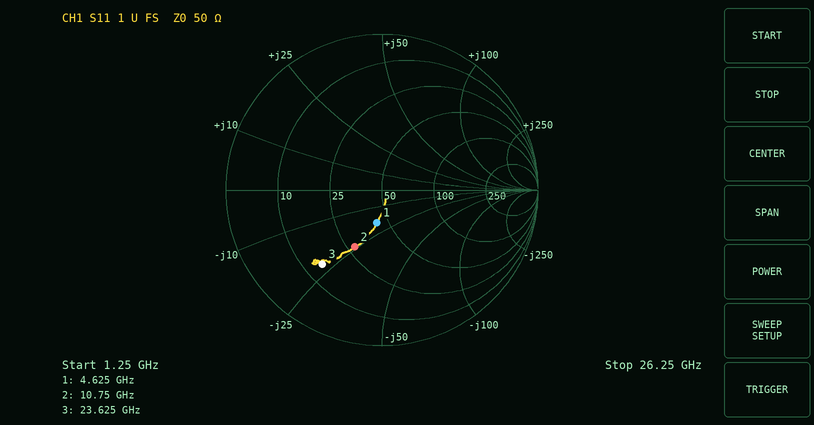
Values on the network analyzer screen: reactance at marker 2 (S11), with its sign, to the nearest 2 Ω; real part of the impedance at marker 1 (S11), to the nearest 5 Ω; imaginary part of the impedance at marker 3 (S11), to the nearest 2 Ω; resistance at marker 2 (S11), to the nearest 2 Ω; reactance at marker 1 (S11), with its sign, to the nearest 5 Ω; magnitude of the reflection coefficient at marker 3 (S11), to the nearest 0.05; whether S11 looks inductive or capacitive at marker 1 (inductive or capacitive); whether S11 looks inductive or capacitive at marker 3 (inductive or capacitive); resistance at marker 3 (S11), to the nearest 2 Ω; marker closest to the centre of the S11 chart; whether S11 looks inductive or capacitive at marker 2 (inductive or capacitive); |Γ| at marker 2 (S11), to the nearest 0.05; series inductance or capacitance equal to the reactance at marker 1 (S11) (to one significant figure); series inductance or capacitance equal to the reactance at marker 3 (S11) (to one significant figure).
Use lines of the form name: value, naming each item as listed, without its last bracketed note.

reactance at marker 2 (S11), with its sign, to the nearest 2 Ω: -24 Ω
real part of the impedance at marker 1 (S11), to the nearest 5 Ω: 45 Ω
imaginary part of the impedance at marker 3 (S11), to the nearest 2 Ω: -22 Ω
resistance at marker 2 (S11), to the nearest 2 Ω: 28 Ω
reactance at marker 1 (S11), with its sign, to the nearest 5 Ω: -20 Ω
magnitude of the reflection coefficient at marker 3 (S11), to the nearest 0.05: 0.60
whether S11 looks inductive or capacitive at marker 1: capacitive
whether S11 looks inductive or capacitive at marker 3: capacitive
resistance at marker 3 (S11), to the nearest 2 Ω: 14 Ω
marker closest to the centre of the S11 chart: marker 1
whether S11 looks inductive or capacitive at marker 2: capacitive
|Γ| at marker 2 (S11), to the nearest 0.05: 0.40
series inductance or capacitance equal to the reactance at marker 1 (S11): 2 pF
series inductance or capacitance equal to the reactance at marker 3 (S11): 300 fF
